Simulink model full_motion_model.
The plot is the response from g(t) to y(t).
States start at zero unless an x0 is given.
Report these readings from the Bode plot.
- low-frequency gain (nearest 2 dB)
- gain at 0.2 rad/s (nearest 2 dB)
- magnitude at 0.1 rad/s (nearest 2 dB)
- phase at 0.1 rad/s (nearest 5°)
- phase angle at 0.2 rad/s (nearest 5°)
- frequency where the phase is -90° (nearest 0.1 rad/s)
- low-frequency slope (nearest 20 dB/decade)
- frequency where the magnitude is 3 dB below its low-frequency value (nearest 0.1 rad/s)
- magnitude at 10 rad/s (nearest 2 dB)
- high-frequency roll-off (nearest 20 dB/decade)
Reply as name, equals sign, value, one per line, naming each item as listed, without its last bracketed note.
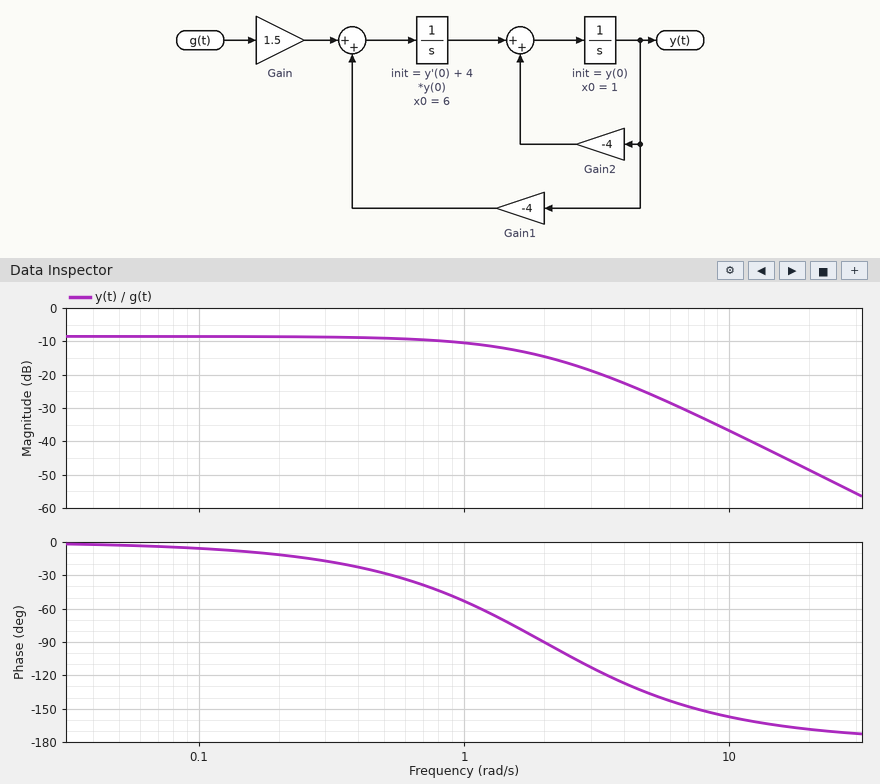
low-frequency gain = -8 dB
gain at 0.2 rad/s = -8 dB
magnitude at 0.1 rad/s = -8 dB
phase at 0.1 rad/s = -5°
phase angle at 0.2 rad/s = -10°
frequency where the phase is -90° = 2.0 rad/s
low-frequency slope = 0 dB/decade
frequency where the magnitude is 3 dB below its low-frequency value = 1.3 rad/s
magnitude at 10 rad/s = -36 dB
high-frequency roll-off = -40 dB/decade
